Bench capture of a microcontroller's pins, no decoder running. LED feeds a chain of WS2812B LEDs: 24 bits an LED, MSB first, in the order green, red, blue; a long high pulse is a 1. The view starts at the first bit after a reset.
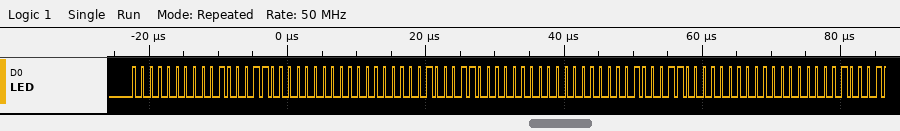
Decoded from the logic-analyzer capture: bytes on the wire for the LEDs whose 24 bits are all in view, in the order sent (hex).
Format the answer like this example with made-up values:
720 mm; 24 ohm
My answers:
00 23 00 00 23 00 00 23 00
